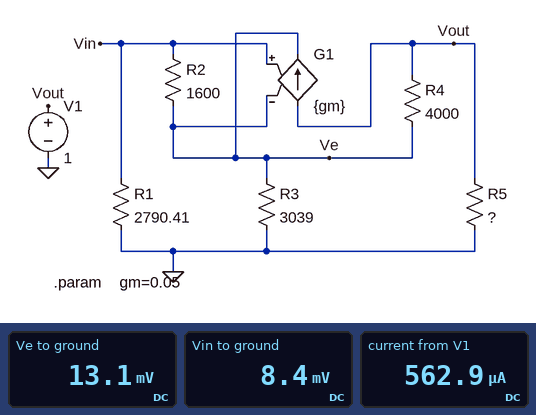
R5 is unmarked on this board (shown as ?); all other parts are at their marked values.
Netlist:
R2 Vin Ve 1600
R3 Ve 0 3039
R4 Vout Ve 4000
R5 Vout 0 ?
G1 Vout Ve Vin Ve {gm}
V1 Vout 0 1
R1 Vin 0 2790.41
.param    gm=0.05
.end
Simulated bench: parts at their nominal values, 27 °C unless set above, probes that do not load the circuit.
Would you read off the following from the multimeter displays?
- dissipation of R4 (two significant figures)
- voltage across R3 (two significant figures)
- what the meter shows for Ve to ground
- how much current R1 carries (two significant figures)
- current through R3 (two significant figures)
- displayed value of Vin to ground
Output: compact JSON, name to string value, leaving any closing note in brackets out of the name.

{"dissipation of R4": "240 µW", "voltage across R3": "13 mV", "what the meter shows for Ve to ground": "13.1 mV", "how much current R1 carries": "3.0 µA", "current through R3": "4.3 µA", "displayed value of Vin to ground": "8.4 mV"}
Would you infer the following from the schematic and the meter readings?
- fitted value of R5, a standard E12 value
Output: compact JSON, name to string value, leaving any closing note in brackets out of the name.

{"fitted value of R5, a standard E12 value": "1.8 kΩ"}
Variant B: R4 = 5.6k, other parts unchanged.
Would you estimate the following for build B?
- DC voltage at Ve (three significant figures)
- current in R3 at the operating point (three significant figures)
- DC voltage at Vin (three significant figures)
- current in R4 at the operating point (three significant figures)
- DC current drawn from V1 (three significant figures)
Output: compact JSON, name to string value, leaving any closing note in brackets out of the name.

{"DC voltage at Ve": "9.42 mV", "current in R3 at the operating point": "3.10 µA", "DC voltage at Vin": "5.99 mV", "current in R4 at the operating point": "177 µA", "DC current drawn from V1": "561 µA"}
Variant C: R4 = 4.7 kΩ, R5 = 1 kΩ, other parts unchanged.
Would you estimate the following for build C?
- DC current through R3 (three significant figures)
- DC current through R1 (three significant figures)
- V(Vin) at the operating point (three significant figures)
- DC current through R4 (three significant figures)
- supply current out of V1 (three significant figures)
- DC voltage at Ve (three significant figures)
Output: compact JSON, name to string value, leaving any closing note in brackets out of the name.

{"DC current through R3": "3.69 µA", "DC current through R1": "2.55 µA", "V(Vin) at the operating point": "7.12 mV", "DC current through R4": "210 µA", "supply current out of V1": "1.01 mA", "DC voltage at Ve": "11.2 mV"}
